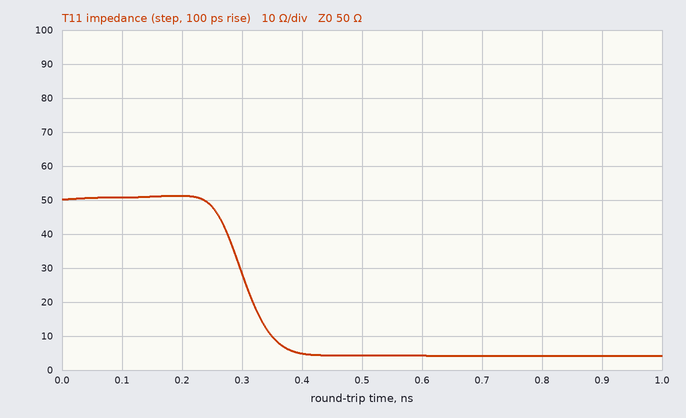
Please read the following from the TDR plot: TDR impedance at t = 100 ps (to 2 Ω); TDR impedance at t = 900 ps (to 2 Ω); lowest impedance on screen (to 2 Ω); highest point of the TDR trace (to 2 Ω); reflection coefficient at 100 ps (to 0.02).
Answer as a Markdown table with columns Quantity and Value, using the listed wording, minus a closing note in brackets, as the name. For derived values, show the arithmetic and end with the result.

| Quantity | Value |
|---|---|
| TDR impedance at t = 100 ps | 50 Ω |
| TDR impedance at t = 900 ps | 4 Ω |
| lowest impedance on screen | 4 Ω |
| highest point of the TDR trace | 52 Ω |
| reflection coefficient at 100 ps | (50 − 50)/(50 + 50) ≈ 0.00 |
